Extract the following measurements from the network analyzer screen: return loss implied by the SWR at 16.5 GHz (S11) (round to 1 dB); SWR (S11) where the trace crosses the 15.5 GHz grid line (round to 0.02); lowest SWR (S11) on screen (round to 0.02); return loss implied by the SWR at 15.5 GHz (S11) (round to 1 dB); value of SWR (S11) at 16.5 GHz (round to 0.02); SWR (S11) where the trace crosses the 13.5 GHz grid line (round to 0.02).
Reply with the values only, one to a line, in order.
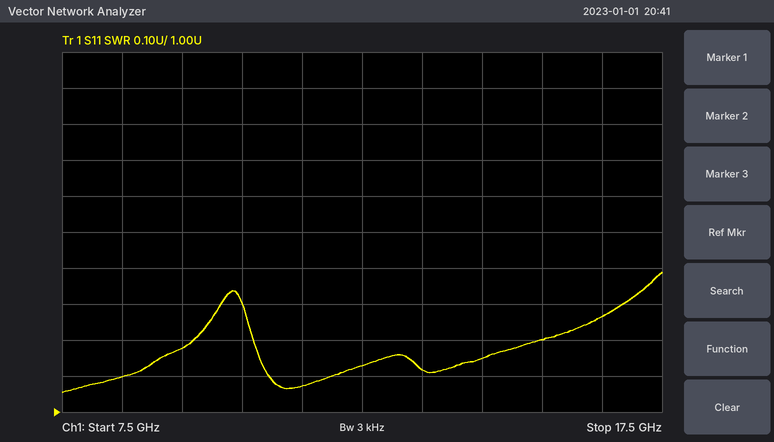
19 dB
1.20
1.06
21 dB
1.26
1.12
